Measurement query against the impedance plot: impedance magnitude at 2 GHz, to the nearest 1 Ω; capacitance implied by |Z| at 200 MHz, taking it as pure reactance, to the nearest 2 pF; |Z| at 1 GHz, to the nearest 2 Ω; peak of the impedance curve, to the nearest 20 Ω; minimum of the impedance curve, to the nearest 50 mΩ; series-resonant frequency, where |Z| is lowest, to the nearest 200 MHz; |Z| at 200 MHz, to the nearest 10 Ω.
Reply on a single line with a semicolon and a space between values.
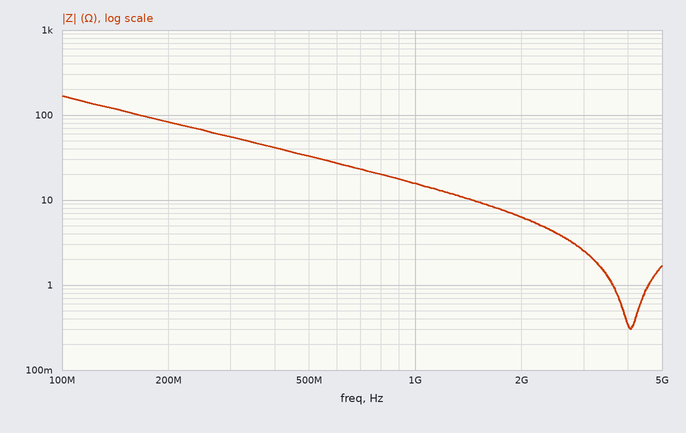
6 Ω; 10 pF; 16 Ω; 160 Ω; 300 mΩ; 4.0 GHz; 80 Ω
